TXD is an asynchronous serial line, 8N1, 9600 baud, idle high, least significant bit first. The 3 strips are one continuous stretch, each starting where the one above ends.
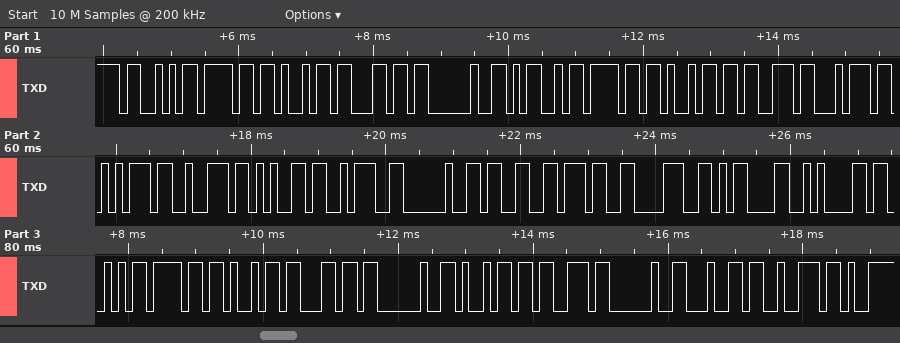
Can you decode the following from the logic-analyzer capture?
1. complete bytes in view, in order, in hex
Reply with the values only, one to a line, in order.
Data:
53 6F 69 6C 20 4D 6F 69 73 74 75 72 65 3A 20 33 37 38 0D 0A 53 6F 69 6C 20 69 73 20 64 72
